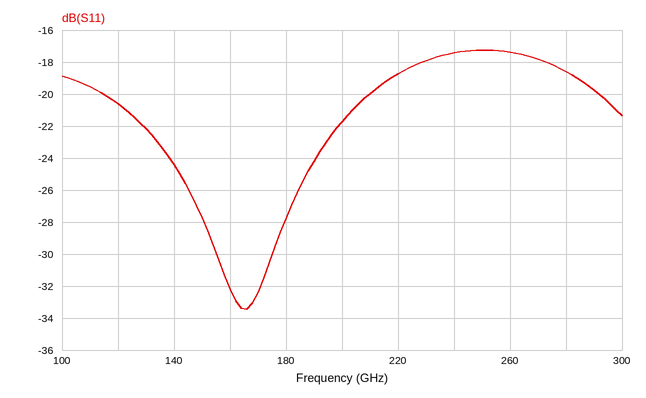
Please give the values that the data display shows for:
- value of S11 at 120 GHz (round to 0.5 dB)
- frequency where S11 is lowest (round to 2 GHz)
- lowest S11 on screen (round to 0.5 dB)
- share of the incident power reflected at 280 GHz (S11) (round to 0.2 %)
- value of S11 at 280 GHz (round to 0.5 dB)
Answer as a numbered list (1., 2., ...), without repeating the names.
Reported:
1. -20.5 dB
2. 166 GHz
3. -33.5 dB
4. 1.4 %
5. -18.5 dB
